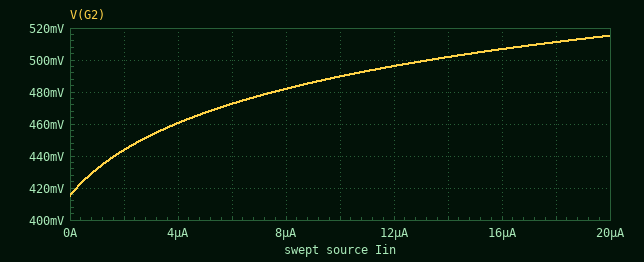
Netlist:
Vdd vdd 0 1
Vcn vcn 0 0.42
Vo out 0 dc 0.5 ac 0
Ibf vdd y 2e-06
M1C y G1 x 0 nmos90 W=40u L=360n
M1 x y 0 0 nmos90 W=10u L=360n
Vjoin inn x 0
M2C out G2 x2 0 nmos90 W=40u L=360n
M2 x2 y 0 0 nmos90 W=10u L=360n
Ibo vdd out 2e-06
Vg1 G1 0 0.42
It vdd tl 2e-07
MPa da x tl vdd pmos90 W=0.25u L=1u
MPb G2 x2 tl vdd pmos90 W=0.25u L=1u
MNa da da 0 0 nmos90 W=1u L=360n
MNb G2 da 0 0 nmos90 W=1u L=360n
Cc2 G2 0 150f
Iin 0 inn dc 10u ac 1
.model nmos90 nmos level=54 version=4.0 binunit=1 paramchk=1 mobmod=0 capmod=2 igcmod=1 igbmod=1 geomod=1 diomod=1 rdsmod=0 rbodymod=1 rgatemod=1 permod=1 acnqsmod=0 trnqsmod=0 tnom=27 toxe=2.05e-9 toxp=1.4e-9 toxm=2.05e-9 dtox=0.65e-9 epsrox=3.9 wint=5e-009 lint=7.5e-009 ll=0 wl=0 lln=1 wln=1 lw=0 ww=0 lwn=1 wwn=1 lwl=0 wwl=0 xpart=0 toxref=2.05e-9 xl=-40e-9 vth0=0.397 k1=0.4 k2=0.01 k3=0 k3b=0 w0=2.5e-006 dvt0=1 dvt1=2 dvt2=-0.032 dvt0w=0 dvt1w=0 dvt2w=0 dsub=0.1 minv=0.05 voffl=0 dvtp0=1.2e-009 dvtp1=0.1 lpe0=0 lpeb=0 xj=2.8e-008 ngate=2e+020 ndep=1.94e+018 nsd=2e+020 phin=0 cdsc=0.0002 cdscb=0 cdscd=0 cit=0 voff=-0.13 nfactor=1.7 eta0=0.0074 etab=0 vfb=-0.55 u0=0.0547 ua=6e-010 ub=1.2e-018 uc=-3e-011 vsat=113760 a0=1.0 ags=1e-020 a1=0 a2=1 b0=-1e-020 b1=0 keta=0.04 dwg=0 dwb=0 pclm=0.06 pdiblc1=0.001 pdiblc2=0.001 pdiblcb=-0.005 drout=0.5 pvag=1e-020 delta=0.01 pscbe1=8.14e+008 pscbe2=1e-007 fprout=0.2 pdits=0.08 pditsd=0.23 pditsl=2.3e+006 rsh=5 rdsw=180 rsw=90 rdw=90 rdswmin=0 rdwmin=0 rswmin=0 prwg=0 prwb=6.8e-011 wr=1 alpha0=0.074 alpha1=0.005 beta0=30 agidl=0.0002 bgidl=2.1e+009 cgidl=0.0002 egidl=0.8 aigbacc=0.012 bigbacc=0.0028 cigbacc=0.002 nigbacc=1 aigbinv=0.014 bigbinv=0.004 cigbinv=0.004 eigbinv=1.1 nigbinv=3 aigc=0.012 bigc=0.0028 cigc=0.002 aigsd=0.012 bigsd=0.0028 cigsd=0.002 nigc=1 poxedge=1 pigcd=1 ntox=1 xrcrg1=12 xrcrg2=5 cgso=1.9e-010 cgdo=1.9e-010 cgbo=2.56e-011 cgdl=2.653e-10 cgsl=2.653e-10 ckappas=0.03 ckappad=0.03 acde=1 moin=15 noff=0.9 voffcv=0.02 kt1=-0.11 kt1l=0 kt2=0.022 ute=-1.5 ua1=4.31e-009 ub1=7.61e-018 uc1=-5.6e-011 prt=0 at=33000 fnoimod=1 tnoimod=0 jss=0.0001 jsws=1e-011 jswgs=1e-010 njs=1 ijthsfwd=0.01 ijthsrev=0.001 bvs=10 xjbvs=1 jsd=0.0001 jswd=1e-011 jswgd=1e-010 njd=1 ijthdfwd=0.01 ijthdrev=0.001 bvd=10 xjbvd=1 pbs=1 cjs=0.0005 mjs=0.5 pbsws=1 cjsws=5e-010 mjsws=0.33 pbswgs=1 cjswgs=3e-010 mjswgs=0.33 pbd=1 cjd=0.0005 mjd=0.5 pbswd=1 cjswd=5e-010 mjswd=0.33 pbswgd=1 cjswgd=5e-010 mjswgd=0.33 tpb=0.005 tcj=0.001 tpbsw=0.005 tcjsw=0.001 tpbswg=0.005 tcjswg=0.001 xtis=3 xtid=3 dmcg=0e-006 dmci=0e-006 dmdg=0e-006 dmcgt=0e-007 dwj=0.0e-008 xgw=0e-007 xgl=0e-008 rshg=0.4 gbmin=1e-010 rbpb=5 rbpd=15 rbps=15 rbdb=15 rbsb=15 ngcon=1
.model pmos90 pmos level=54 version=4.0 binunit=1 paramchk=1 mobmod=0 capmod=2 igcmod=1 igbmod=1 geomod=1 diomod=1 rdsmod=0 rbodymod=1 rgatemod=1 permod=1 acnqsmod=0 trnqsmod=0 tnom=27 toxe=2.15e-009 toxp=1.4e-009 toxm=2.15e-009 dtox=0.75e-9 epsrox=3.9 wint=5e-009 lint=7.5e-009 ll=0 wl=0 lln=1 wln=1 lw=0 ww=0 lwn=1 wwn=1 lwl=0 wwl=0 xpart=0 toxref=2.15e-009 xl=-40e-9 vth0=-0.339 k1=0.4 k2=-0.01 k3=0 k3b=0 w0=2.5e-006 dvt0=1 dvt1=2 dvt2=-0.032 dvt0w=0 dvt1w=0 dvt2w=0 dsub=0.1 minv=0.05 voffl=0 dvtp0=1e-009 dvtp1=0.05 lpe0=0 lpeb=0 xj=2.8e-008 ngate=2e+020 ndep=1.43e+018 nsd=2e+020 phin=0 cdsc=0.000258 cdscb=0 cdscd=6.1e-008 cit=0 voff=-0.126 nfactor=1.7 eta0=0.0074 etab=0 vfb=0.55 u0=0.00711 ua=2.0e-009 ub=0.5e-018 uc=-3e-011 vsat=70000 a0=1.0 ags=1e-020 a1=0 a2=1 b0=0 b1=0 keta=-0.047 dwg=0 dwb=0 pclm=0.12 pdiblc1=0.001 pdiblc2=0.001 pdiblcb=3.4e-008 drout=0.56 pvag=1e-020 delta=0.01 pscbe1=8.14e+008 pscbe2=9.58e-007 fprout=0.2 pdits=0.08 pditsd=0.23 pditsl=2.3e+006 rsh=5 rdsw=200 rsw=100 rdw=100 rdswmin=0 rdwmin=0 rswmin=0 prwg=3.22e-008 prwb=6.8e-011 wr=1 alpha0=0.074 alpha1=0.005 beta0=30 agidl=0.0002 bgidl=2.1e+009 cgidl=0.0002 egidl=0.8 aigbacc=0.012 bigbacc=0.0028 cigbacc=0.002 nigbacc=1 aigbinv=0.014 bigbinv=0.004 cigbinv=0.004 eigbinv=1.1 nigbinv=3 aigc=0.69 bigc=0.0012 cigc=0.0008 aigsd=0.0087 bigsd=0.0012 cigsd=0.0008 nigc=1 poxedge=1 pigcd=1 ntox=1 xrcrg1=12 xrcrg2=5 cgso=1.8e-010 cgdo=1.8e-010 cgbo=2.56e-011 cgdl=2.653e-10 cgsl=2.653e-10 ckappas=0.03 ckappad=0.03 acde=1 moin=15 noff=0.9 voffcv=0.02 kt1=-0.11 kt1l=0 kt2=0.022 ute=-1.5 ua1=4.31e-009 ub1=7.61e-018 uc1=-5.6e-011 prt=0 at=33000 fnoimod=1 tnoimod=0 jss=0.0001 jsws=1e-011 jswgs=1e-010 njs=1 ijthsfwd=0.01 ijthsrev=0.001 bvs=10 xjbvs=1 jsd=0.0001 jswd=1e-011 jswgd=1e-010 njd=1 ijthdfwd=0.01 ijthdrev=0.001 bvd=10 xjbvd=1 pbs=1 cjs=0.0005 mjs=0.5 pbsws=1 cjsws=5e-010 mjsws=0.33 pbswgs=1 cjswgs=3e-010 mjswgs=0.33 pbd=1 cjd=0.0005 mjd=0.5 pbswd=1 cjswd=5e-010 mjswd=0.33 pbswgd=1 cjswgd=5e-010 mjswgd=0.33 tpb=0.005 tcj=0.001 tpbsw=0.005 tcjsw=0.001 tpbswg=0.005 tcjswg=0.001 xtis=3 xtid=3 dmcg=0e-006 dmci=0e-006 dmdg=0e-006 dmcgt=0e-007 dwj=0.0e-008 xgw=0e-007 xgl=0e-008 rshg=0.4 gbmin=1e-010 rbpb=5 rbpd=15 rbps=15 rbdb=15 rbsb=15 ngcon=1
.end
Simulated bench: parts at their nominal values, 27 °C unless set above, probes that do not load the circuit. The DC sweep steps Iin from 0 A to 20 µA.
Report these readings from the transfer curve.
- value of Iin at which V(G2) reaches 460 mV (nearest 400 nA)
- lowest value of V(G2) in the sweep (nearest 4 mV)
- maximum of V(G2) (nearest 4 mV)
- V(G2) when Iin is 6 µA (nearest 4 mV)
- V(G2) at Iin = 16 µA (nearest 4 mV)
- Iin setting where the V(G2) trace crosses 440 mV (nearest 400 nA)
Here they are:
4.0 µA
416 mV
516 mV
472 mV
508 mV
1.6 µA
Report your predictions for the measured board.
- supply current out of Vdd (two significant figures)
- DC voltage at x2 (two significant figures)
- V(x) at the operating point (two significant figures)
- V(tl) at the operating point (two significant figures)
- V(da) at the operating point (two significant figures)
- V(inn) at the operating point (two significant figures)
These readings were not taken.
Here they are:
4.2 µA
170 mV
180 mV
660 mV
230 mV
180 mV
